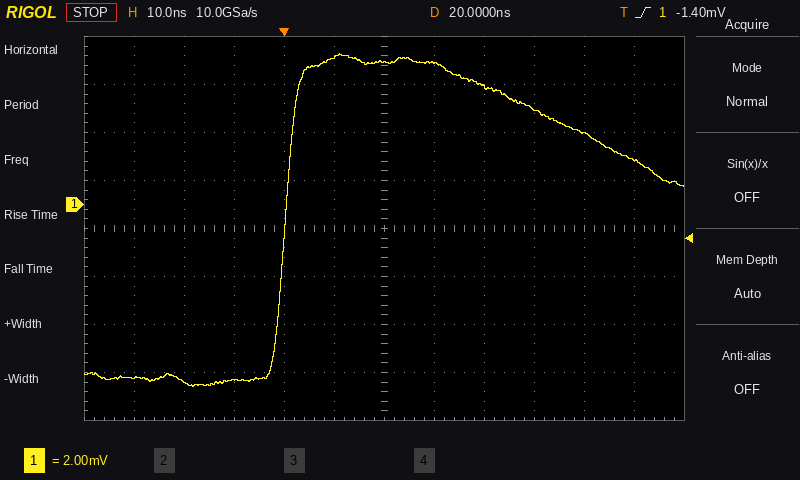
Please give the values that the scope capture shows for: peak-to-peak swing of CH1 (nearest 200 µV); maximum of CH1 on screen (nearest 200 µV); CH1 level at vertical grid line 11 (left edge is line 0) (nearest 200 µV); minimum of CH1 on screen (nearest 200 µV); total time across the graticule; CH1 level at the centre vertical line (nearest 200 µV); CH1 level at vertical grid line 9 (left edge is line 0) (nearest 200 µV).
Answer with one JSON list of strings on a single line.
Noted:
["13.8 mV", "6.2 mV", "1.8 mV", "-7.6 mV", "120 ns", "6.0 mV", "4.0 mV"]
